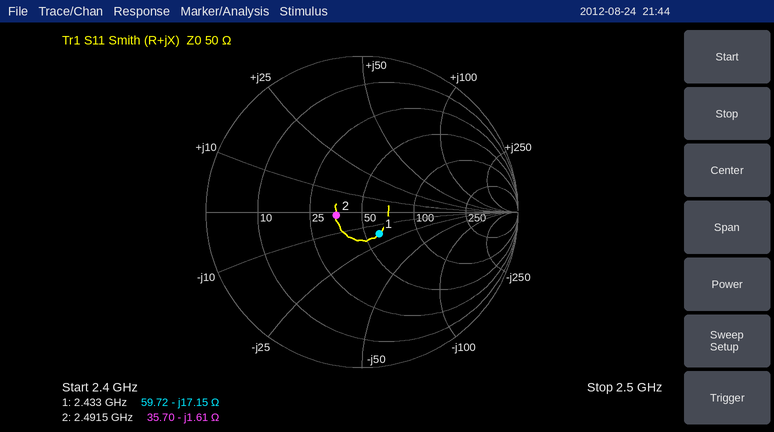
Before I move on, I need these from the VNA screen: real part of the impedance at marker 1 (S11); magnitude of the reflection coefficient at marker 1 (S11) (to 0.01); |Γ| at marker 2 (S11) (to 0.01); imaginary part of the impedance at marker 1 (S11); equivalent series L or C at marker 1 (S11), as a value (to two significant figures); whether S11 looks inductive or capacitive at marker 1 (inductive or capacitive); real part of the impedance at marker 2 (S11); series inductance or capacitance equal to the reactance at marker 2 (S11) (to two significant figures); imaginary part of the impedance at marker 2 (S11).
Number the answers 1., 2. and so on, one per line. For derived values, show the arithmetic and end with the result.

1. 59.72 Ω
2. 0.18
3. 0.17
4. -17.15 Ω
5. C = 1/(2π × 2.433 GHz × 17.15 Ω) ≈ 3.8 pF
6. capacitive
7. 35.70 Ω
8. C = 1/(2π × 2.4915 GHz × 1.61 Ω) ≈ 40 pF
9. -1.61 Ω
